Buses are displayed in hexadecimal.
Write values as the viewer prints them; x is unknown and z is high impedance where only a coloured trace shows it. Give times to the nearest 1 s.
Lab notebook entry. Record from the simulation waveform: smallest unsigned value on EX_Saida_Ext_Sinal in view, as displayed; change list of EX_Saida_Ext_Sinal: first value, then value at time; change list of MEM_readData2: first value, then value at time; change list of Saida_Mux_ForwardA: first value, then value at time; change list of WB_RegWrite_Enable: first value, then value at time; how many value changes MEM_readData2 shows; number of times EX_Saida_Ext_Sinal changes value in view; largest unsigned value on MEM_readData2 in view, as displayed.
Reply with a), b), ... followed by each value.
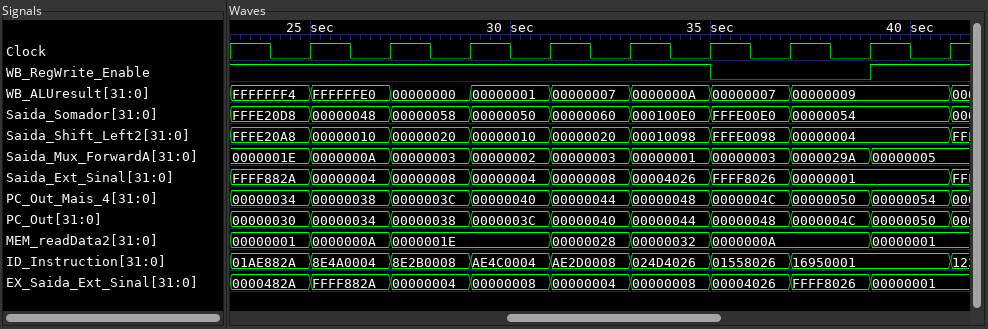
a) 00000001
b) 0000482A, FFFF882A at 25 s, 00000004 at 27 s, 00000008 at 29 s, 00000004 at 31 s, 00000008 at 33 s, 00004026 at 35 s, FFFF8026 at 37 s, 00000001 at 39 s
c) 00000001, 0000000A at 25 s, 0000001E at 27 s, 00000028 at 31 s, 00000032 at 33 s, 0000000A at 35 s, 00000001 at 39 s
d) 0000001E, 0000000A at 25 s, 00000003 at 27 s, 00000002 at 29 s, 00000003 at 31 s, 00000001 at 33 s, 00000003 at 35 s, 0000029A at 37 s, 00000005 at 39 s
e) 1, 0 at 35 s, 1 at 39 s
f) 6
g) 8
h) 00000032
